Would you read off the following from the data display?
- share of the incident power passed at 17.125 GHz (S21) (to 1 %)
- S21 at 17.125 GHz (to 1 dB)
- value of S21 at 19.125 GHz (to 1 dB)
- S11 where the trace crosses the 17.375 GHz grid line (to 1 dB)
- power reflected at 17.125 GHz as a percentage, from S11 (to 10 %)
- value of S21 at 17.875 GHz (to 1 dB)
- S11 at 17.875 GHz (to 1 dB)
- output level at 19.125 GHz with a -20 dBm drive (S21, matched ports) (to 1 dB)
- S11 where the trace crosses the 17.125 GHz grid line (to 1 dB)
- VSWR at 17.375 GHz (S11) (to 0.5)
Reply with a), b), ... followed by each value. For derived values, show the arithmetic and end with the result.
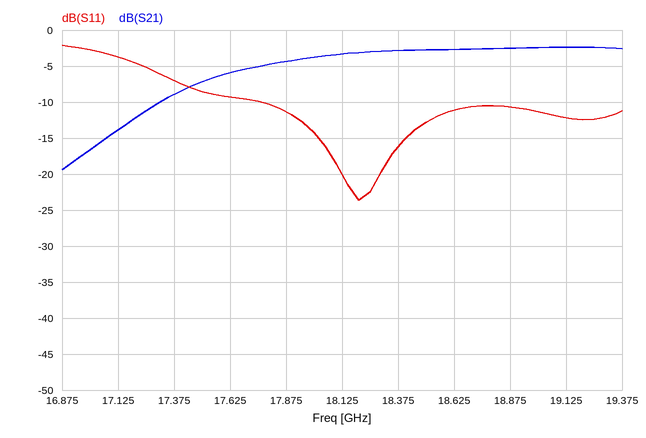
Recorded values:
a) 10^(-14/10) ≈ 4 %
b) -14 dB
c) -2 dB
d) -7 dB
e) 10^(-4/10) ≈ 40 %
f) -4 dB
g) -11 dB
h) -20 dBm + (-2 dB) = -22 dBm
i) -4 dB
j) |Γ| = 10^(-7/20) = 0.4467; VSWR = (1 + 0.4467)/(1 − 0.4467) ≈ 2.61, so 2.5 to the nearest 0.5
